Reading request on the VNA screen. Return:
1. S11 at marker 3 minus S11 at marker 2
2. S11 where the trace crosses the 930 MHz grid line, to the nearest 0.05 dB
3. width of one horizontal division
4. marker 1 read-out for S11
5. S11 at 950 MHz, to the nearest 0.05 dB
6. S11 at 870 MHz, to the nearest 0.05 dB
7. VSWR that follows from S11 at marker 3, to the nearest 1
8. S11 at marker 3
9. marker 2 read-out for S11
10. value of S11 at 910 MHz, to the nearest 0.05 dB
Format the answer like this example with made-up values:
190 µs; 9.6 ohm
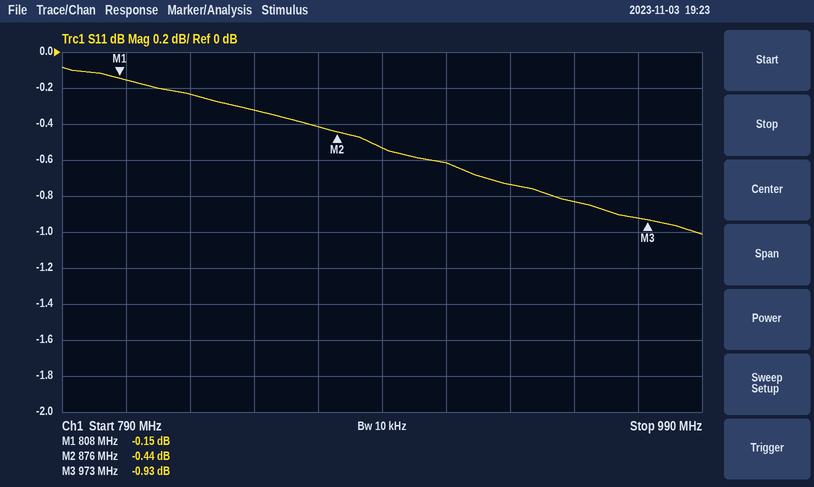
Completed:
-0.49 dB; -0.75 dB; 20 MHz; -0.15 dB; -0.85 dB; -0.40 dB; 19; -0.93 dB; -0.44 dB; -0.60 dB
